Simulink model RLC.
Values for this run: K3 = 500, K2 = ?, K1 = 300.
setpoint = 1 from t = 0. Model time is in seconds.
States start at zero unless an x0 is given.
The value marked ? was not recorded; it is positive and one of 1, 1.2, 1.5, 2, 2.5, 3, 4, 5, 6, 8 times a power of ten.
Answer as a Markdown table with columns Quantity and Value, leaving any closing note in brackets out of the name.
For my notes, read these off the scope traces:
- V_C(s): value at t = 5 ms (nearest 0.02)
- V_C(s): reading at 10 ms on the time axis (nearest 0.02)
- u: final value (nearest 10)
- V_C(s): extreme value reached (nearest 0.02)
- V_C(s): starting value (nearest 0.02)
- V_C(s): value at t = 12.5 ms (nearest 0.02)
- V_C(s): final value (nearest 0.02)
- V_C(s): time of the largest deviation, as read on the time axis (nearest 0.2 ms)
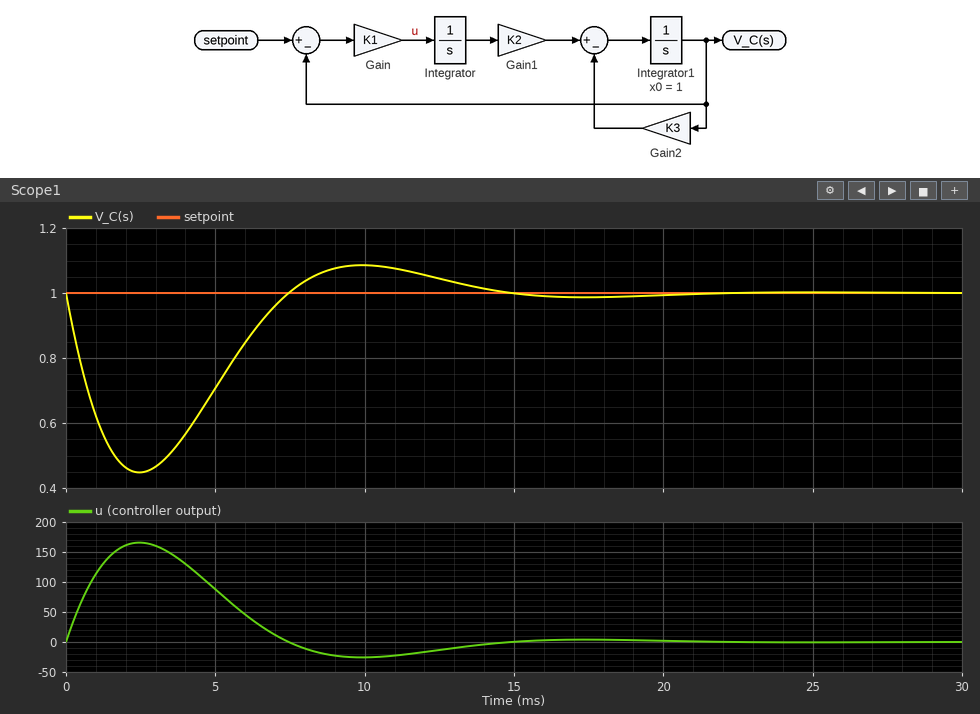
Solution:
| Quantity | Value |
|---|---|
| V_C(s): value at t = 5 ms | 0.70 |
| V_C(s): reading at 10 ms on the time axis | 1.08 |
| u: final value | 0 |
| V_C(s): extreme value reached | 0.44 |
| V_C(s): starting value | 1.00 |
| V_C(s): value at t = 12.5 ms | 1.04 |
| V_C(s): final value | 1.00 |
| V_C(s): time of the largest deviation, as read on the time axis | 2.4 ms |
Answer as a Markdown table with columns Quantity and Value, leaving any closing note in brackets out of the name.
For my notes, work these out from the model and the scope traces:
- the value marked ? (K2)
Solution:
| Quantity | Value |
|---|---|
| the value marked ? | 800 |
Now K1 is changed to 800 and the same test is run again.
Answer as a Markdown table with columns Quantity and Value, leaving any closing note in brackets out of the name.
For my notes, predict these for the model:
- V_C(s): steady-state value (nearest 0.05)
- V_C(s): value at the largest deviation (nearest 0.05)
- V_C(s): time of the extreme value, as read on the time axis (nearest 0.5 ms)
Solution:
| Quantity | Value |
|---|---|
| V_C(s): steady-state value | 1.00 |
| V_C(s): value at the largest deviation | 0.60 |
| V_C(s): time of the extreme value, as read on the time axis | 1.5 ms |
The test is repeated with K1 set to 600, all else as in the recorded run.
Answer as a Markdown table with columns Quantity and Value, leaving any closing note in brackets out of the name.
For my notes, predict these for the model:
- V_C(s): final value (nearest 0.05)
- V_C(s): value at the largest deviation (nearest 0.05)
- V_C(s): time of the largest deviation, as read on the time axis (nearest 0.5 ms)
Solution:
| Quantity | Value |
|---|---|
| V_C(s): final value | 1.00 |
| V_C(s): value at the largest deviation | 0.55 |
| V_C(s): time of the largest deviation, as read on the time axis | 2.0 ms |
